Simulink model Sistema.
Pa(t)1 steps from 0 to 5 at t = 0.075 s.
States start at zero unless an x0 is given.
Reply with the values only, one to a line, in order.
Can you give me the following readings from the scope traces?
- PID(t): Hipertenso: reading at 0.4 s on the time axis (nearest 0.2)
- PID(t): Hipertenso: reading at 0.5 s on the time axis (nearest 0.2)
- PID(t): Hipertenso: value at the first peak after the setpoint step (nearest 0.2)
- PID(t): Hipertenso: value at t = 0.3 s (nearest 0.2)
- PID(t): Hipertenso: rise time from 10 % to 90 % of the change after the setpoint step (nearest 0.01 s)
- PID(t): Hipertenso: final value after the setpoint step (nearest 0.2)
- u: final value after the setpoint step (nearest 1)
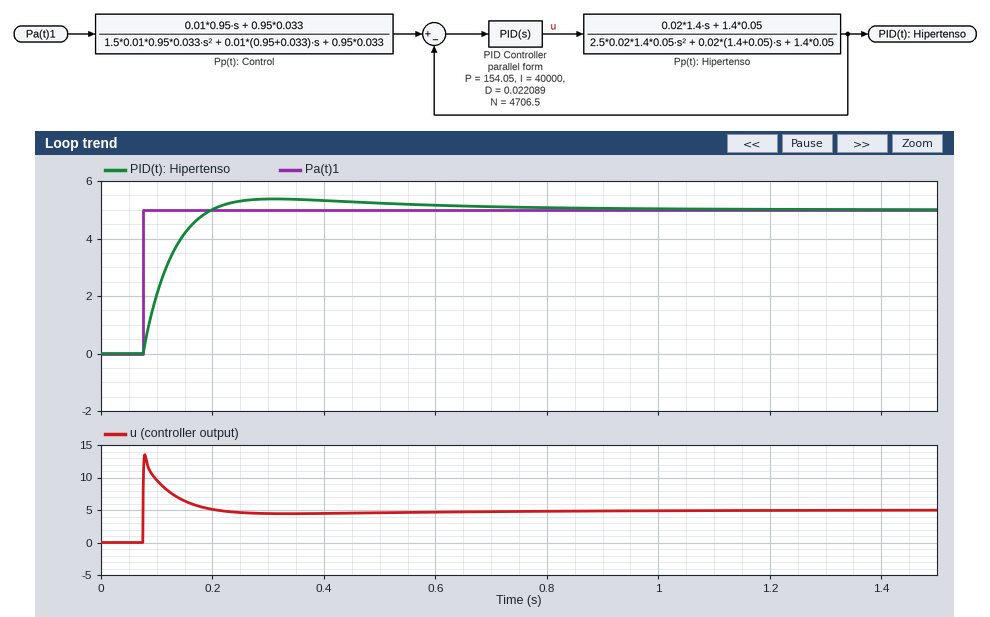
5.4
5.2
5.4
5.4
0.08 s
5.0
5
